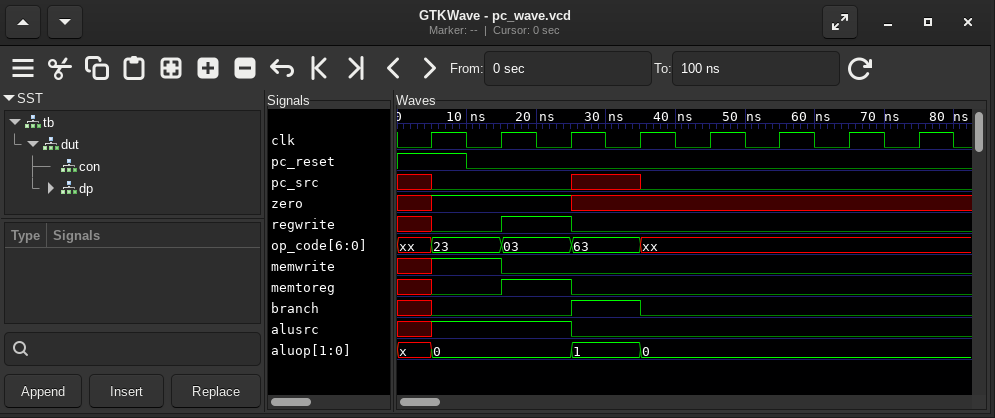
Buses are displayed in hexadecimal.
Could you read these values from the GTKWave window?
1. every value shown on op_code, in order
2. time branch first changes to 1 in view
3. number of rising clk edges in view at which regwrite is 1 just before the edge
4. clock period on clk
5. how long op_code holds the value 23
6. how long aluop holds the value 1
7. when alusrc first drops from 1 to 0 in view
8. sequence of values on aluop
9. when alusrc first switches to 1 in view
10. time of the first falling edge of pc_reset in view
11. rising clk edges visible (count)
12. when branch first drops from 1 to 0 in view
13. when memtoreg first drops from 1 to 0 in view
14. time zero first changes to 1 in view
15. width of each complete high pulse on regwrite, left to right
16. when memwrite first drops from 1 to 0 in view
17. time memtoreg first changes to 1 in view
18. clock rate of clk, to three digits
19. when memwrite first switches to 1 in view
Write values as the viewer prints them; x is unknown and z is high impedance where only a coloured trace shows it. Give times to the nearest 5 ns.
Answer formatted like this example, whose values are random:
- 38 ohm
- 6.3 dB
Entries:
- xx, 23, 03, 63, xx
- 25 ns
- 1
- 10 ns
- 10 ns
- 10 ns
- 25 ns
- x, 0, 1, 0
- 5 ns
- 10 ns
- 8
- 35 ns
- 25 ns
- 5 ns
- 10 ns
- 15 ns
- 15 ns
- 100 MHz
- 5 ns
